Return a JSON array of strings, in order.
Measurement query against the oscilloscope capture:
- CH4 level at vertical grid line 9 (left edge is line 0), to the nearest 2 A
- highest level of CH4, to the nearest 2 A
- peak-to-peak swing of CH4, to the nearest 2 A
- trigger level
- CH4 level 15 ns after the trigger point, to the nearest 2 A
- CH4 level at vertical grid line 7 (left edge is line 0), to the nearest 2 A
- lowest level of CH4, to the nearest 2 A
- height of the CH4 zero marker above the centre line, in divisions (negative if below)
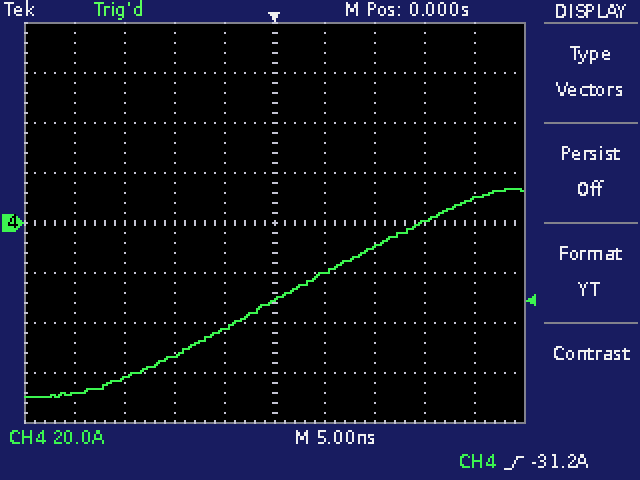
["10 A", "14 A", "84 A", "-31.2 A", "0 A", "-10 A", "-70 A", "0.0 div"]
